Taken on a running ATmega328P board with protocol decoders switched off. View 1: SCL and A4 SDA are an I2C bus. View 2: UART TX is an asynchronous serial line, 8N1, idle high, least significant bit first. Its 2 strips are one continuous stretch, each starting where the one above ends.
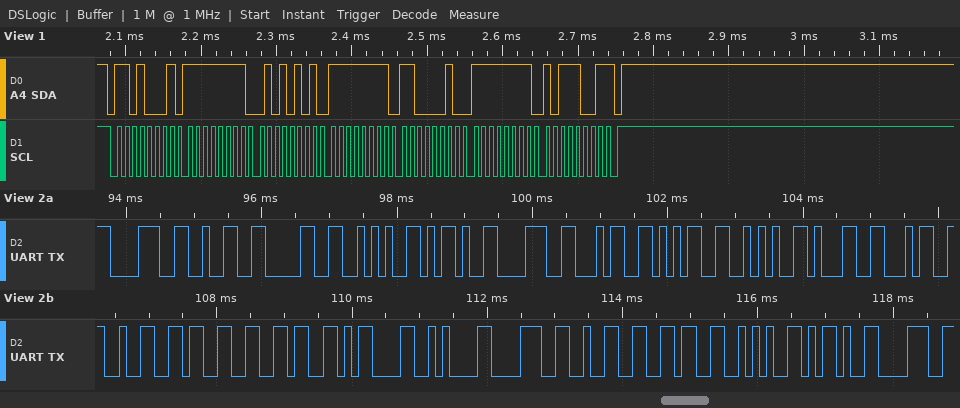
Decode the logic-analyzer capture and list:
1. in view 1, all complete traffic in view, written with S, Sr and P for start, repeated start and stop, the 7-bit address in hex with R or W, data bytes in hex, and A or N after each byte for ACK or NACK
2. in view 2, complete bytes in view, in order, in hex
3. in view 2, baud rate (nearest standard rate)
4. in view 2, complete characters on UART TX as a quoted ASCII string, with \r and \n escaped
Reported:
S 68R A FF A 55 A FF A C2 A FF A B9 N P
0x38 0x32 0x30 0x2A 0x2D 0x38 0x34 0x35 0x2A 0x31 0x34 0x32 0x33 0x36 0x0D 0x0A 0x38 0x32 0x36 0x2A 0x2D 0x38
9600 baud
"820*-845*14236\r\n826*-8"
